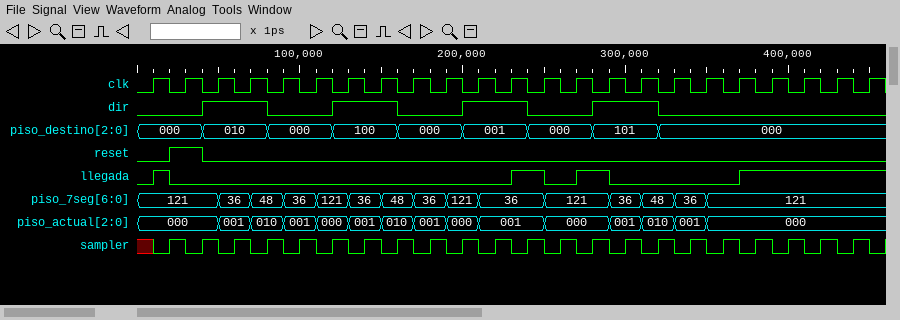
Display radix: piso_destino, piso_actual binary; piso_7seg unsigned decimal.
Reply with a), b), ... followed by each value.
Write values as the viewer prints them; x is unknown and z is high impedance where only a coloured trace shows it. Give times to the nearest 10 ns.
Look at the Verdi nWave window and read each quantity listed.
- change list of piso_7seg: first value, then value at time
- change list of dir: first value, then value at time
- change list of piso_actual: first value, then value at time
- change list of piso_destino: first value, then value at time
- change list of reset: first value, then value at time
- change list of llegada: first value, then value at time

a) 121, 36 at 50 ns, 48 at 70 ns, 36 at 90 ns, 121 at 110 ns, 36 at 130 ns, 48 at 150 ns, 36 at 170 ns, 121 at 190 ns, 36 at 210 ns, 121 at 250 ns, 36 at 290 ns, 48 at 310 ns, 36 at 330 ns, 121 at 350 ns
b) 0, 1 at 40 ns, 0 at 80 ns, 1 at 120 ns, 0 at 160 ns, 1 at 200 ns, 0 at 240 ns, 1 at 280 ns, 0 at 320 ns
c) 000, 001 at 50 ns, 010 at 70 ns, 001 at 90 ns, 000 at 110 ns, 001 at 130 ns, 010 at 150 ns, 001 at 170 ns, 000 at 190 ns, 001 at 210 ns, 000 at 250 ns, 001 at 290 ns, 010 at 310 ns, 001 at 330 ns, 000 at 350 ns
d) 000, 010 at 40 ns, 000 at 80 ns, 100 at 120 ns, 000 at 160 ns, 001 at 200 ns, 000 at 240 ns, 101 at 280 ns, 000 at 320 ns
e) 0, 1 at 20 ns, 0 at 40 ns
f) 0, 1 at 10 ns, 0 at 20 ns, 1 at 230 ns, 0 at 250 ns, 1 at 270 ns, 0 at 290 ns, 1 at 370 ns
